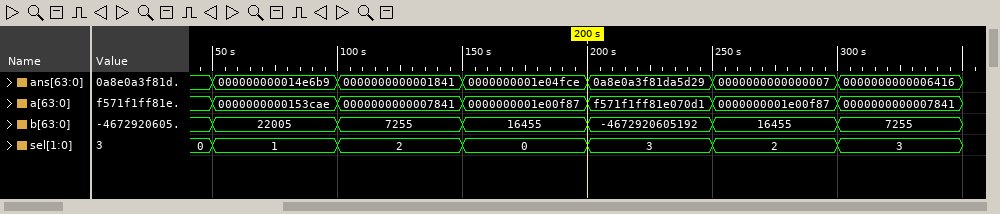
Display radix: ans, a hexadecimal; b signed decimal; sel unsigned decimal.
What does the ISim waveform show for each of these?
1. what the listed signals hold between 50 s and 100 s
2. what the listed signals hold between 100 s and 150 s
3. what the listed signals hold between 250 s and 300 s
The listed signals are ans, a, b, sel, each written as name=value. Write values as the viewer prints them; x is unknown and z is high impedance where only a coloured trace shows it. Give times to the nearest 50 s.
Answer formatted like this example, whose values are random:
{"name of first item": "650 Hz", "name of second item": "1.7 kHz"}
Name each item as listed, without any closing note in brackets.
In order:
{"what the listed signals hold between 50 s and 100 s": "ans=000000000014e6b9, a=0000000000153cae, b=22005, sel=1", "what the listed signals hold between 100 s and 150 s": "ans=0000000000001841, a=0000000000007841, b=7255, sel=2", "what the listed signals hold between 250 s and 300 s": "ans=0000000000000007, a=0000000001e00f87, b=16455, sel=2"}
